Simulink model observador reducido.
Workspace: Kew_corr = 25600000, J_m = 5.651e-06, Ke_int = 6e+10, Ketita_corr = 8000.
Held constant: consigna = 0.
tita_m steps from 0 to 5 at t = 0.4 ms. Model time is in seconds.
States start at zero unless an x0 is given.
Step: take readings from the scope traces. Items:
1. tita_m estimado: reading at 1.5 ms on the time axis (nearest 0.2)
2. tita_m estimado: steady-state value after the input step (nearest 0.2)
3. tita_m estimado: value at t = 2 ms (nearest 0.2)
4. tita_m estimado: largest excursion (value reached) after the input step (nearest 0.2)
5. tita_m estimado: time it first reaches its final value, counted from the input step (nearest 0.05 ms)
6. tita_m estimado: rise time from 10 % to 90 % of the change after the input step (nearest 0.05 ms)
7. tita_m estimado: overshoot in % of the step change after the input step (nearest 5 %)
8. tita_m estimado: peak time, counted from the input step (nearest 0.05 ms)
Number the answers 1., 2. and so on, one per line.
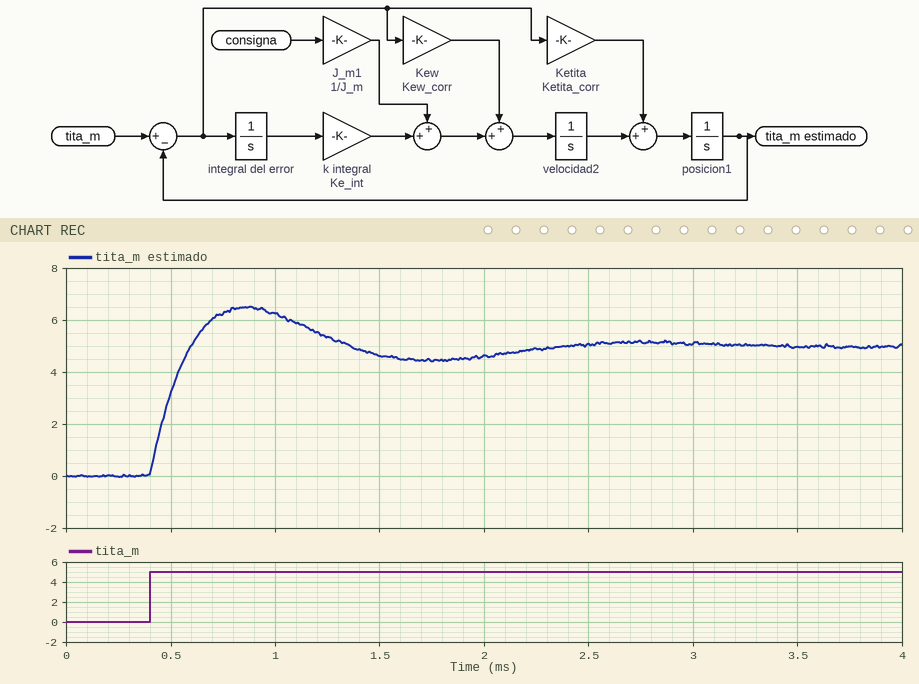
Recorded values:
1. 4.6
2. 5.0
3. 4.6
4. 6.4
5. 0.20 ms
6. 0.15 ms
7. 30 %
8. 0.45 ms
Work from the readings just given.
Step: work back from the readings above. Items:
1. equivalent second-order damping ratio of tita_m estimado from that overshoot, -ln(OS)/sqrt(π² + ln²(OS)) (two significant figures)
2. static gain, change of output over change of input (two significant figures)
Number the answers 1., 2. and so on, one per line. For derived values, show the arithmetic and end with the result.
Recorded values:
1. ln(0.3) = -1.204; 1.204 / sqrt(9.870 + 1.450) = 0.36
2. (5 - 0) / (5 - 0) = 1.0
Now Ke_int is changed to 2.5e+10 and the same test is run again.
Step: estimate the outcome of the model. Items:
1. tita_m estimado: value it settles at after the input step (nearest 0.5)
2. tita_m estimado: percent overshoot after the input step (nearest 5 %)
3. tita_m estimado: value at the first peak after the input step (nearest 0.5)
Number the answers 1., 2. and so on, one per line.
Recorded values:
1. 5.0
2. 25 %
3. 6.0
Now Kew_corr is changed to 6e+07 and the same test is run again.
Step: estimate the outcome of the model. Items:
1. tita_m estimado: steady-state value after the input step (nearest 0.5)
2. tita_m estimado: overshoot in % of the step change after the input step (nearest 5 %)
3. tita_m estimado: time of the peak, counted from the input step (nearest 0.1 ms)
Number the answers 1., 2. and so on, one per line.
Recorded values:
1. 5.0
2. 35 %
3. 0.3 ms
